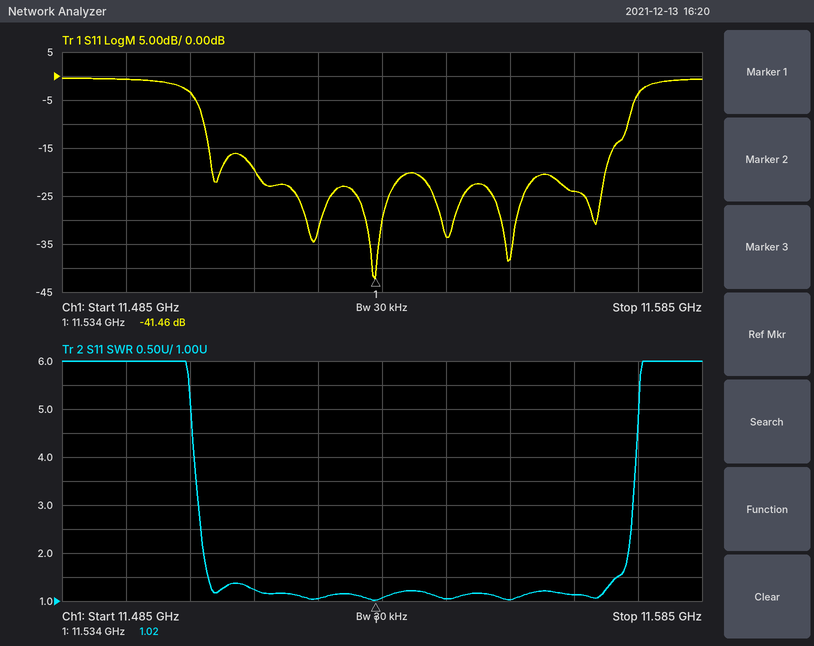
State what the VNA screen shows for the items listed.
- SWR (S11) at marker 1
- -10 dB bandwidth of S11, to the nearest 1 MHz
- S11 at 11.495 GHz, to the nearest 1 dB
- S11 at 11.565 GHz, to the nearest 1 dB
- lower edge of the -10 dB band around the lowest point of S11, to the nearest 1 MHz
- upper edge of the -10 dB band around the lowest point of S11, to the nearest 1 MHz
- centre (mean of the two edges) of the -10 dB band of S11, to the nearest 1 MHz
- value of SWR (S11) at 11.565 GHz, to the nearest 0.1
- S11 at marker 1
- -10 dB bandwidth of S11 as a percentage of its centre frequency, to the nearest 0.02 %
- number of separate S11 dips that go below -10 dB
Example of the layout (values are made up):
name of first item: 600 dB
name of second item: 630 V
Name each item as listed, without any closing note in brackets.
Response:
SWR (S11) at marker 1: 1.02
-10 dB bandwidth of S11, to the nearest 1 MHz: 66 MHz
S11 at 11.495 GHz, to the nearest 1 dB: -1 dB
S11 at 11.565 GHz, to the nearest 1 dB: -24 dB
lower edge of the -10 dB band around the lowest point of S11, to the nearest 1 MHz: 11.507 GHz
upper edge of the -10 dB band around the lowest point of S11, to the nearest 1 MHz: 11.573 GHz
centre (mean of the two edges) of the -10 dB band of S11, to the nearest 1 MHz: 11.540 GHz
value of SWR (S11) at 11.565 GHz, to the nearest 0.1: 1.1
S11 at marker 1: -41.46 dB
-10 dB bandwidth of S11 as a percentage of its centre frequency, to the nearest 0.02 %: 0.58 %
number of separate S11 dips that go below -10 dB: 6
